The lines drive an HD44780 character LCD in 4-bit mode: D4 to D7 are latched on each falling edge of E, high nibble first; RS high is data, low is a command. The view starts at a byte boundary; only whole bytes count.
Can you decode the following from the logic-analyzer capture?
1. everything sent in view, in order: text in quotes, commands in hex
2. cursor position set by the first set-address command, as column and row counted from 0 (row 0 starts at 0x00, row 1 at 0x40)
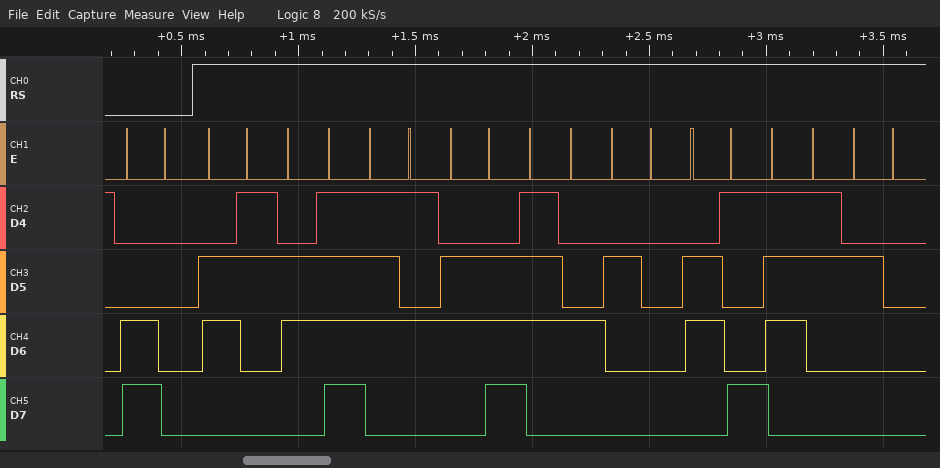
0xC0 "count is "
column 0, row 1
